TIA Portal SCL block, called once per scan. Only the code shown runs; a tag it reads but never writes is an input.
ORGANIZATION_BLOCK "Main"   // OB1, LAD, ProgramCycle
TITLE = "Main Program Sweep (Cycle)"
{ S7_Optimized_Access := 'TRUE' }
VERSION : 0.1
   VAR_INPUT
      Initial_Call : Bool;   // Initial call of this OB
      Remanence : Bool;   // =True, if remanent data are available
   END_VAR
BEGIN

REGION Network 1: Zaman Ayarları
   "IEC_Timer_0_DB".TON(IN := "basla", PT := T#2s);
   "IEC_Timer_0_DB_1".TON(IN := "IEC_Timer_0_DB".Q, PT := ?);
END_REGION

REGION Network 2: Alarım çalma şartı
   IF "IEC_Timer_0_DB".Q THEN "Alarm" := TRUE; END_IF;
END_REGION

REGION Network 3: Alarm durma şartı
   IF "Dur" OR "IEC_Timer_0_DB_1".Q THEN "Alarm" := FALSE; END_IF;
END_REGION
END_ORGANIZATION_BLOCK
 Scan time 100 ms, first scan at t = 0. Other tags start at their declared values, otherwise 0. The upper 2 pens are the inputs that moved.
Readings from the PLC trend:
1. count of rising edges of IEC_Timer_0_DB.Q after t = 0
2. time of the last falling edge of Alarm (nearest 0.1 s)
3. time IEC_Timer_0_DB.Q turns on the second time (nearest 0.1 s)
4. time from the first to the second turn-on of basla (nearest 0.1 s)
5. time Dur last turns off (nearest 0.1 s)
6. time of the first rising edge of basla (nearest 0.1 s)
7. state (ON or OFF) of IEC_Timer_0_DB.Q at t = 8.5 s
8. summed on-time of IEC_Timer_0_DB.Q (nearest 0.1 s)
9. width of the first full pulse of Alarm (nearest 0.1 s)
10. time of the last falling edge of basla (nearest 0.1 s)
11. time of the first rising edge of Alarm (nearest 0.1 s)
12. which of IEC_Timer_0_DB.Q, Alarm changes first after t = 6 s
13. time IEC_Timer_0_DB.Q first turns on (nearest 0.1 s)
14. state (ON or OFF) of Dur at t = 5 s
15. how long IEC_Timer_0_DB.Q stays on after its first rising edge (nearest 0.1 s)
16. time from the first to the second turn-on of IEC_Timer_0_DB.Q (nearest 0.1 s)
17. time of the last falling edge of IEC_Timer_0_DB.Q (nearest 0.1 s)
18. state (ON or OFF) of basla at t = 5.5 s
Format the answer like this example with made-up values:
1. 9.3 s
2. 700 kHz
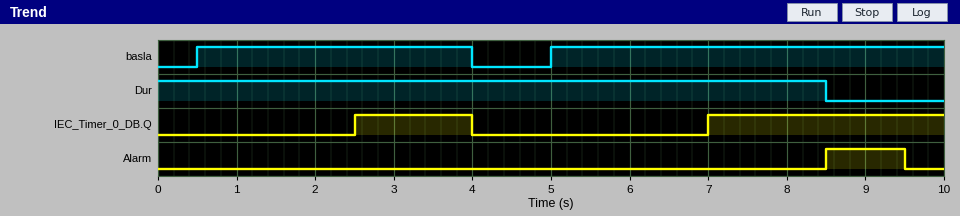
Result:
1. 2
2. 9.5 s
3. 7.0 s
4. 4.5 s
5. 8.5 s
6. 0.5 s
7. ON
8. 4.5 s
9. 1.0 s
10. 4.0 s
11. 8.5 s
12. IEC_Timer_0_DB.Q
13. 2.5 s
14. ON
15. 1.5 s
16. 4.5 s
17. 4.0 s
18. ON
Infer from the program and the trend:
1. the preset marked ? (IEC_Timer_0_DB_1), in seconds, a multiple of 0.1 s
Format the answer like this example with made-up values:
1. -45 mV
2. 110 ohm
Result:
1. 2.5 s
